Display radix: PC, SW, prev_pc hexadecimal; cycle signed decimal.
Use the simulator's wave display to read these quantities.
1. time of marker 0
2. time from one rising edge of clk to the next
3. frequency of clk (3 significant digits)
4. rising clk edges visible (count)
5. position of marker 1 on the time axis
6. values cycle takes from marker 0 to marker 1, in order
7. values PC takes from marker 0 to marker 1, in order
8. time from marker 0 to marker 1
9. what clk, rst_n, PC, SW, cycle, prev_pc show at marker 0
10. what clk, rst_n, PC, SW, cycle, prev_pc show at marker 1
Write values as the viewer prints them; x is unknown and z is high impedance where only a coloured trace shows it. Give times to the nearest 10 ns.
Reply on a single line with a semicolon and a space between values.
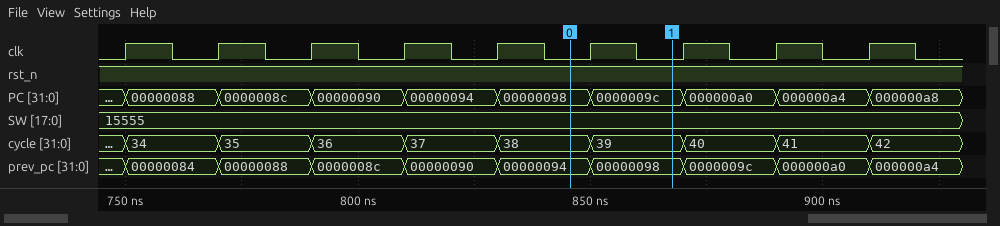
850 ns; 20 ns; 50.0 MHz; 9; 870 ns; 38, 39; 00000098, 0000009c; 20 ns; clk=0, rst_n=1, PC=00000098, SW=15555, cycle=38, prev_pc=00000094; clk=0, rst_n=1, PC=0000009c, SW=15555, cycle=39, prev_pc=00000098
